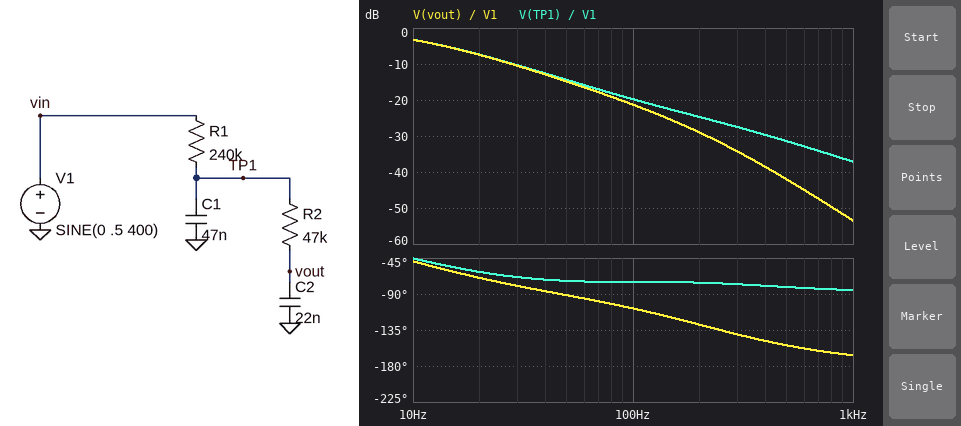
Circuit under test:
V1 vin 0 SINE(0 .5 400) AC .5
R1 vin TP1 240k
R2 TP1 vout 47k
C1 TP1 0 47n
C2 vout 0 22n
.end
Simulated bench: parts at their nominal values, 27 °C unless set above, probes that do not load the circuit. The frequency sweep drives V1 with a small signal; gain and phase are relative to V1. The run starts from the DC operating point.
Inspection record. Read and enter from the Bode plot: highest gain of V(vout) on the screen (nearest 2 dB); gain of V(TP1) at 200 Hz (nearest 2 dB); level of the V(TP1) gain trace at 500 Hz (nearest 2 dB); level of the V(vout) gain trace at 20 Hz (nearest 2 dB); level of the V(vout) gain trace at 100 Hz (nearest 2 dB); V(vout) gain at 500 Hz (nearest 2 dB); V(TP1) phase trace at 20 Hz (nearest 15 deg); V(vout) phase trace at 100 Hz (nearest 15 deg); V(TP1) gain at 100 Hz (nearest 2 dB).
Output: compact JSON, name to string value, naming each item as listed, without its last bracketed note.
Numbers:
{"highest gain of V(vout) on the screen": "-4 dB", "gain of V(TP1) at 200 Hz": "-24 dB", "level of the V(TP1) gain trace at 500 Hz": "-32 dB", "level of the V(vout) gain trace at 20 Hz": "-8 dB", "level of the V(vout) gain trace at 100 Hz": "-22 dB", "V(vout) gain at 500 Hz": "-42 dB", "V(TP1) phase trace at 20 Hz": "-60 deg", "V(vout) phase trace at 100 Hz": "-105 deg", "V(TP1) gain at 100 Hz": "-20 dB"}
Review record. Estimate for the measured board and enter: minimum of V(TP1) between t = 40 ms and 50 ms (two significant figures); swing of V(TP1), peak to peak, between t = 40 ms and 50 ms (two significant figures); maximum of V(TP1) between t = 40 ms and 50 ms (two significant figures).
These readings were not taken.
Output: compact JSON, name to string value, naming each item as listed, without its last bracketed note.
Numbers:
{"minimum of V(TP1) between t = 40 ms and 50 ms": "-16 mV", "swing of V(TP1), peak to peak, between t = 40 ms and 50 ms": "33 mV", "maximum of V(TP1) between t = 40 ms and 50 ms": "17 mV"}
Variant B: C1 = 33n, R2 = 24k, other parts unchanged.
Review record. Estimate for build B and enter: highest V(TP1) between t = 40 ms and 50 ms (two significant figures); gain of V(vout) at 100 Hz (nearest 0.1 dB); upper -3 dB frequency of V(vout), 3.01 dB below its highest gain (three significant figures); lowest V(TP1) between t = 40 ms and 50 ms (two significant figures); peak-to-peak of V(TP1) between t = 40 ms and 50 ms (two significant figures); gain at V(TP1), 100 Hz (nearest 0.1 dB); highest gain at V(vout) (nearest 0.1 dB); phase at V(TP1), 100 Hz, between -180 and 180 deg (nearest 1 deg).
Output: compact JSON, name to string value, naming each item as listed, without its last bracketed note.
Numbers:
{"highest V(TP1) between t = 40 ms and 50 ms": "20 mV", "gain of V(vout) at 100 Hz": "-18.7 dB", "upper -3 dB frequency of V(vout), 3.01 dB below its highest gain": "11.9 Hz", "lowest V(TP1) between t = 40 ms and 50 ms": "-19 mV", "peak-to-peak of V(TP1) between t = 40 ms and 50 ms": "39 mV", "gain at V(TP1), 100 Hz": "-18.3 dB", "highest gain at V(vout)": "0 dB", "phase at V(TP1), 100 Hz, between -180 and 180 deg": "-76 deg"}
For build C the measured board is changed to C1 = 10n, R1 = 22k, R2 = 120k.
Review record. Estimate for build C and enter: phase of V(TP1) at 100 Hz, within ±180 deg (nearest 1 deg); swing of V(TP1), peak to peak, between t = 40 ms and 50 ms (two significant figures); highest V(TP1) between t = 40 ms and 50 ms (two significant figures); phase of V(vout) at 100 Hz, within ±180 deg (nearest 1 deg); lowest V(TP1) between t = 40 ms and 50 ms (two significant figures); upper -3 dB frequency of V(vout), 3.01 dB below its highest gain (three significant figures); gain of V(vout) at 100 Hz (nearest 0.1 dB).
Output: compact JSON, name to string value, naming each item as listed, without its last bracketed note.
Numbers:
{"phase of V(TP1) at 100 Hz, within ±180 deg": "-11 deg", "swing of V(TP1), peak to peak, between t = 40 ms and 50 ms": "760 mV", "highest V(TP1) between t = 40 ms and 50 ms": "380 mV", "phase of V(vout) at 100 Hz, within ±180 deg": "-70 deg", "lowest V(TP1) between t = 40 ms and 50 ms": "-380 mV", "upper -3 dB frequency of V(vout), 3.01 dB below its highest gain": "50.2 Hz", "gain of V(vout) at 100 Hz": "-7.0 dB"}
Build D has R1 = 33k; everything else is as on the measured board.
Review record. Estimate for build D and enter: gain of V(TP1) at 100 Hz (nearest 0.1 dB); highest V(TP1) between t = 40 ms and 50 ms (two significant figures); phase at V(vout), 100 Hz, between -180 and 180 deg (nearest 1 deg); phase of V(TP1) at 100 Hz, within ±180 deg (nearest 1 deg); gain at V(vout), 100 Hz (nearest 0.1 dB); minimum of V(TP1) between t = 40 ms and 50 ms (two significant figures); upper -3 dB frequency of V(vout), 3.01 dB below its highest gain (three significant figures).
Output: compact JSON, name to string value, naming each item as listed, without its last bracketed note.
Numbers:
{"gain of V(TP1) at 100 Hz": "-5.0 dB", "highest V(TP1) between t = 40 ms and 50 ms": "110 mV", "phase at V(vout), 100 Hz, between -180 and 180 deg": "-80 deg", "phase of V(TP1) at 100 Hz, within ±180 deg": "-47 deg", "gain at V(vout), 100 Hz": "-6.5 dB", "minimum of V(TP1) between t = 40 ms and 50 ms": "-110 mV", "upper -3 dB frequency of V(vout), 3.01 dB below its highest gain": "56.0 Hz"}
